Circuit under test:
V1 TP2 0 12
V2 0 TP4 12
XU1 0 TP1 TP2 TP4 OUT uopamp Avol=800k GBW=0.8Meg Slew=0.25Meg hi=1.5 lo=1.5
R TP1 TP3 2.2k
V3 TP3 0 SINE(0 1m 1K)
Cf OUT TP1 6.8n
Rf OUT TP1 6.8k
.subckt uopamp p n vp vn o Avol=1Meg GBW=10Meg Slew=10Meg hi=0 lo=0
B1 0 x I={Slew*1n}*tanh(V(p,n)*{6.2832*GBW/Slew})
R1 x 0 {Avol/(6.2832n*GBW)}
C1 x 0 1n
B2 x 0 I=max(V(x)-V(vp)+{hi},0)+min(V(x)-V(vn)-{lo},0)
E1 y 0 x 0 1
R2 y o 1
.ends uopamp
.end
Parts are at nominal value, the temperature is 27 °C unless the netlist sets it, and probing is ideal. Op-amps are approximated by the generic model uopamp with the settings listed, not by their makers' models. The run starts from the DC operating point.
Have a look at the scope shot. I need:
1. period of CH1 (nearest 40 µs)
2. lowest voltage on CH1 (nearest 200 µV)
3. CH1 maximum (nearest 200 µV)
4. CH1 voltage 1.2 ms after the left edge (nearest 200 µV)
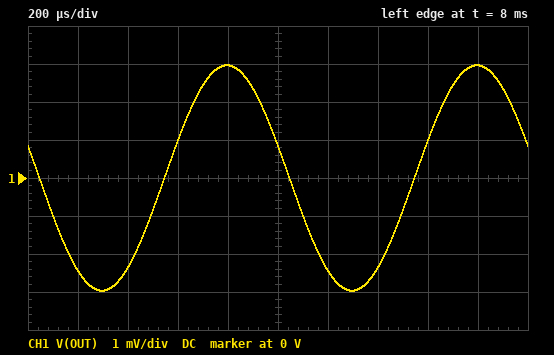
1.00 ms
-3.0 mV
3.0 mV
-2.4 mV
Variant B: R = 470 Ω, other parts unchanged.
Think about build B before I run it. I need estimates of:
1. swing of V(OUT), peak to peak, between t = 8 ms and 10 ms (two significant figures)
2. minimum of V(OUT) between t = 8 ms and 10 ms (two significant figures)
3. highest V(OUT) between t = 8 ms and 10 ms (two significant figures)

28 mV
-14 mV
14 mV
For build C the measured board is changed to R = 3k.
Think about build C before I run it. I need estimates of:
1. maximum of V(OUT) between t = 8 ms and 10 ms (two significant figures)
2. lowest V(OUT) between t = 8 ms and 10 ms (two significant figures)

2.2 mV
-2.2 mV
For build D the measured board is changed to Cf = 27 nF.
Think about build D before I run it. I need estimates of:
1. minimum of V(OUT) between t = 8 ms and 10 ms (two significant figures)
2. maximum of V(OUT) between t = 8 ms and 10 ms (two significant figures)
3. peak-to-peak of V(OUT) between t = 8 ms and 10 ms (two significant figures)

-2.0 mV
2.0 mV
4.0 mV
